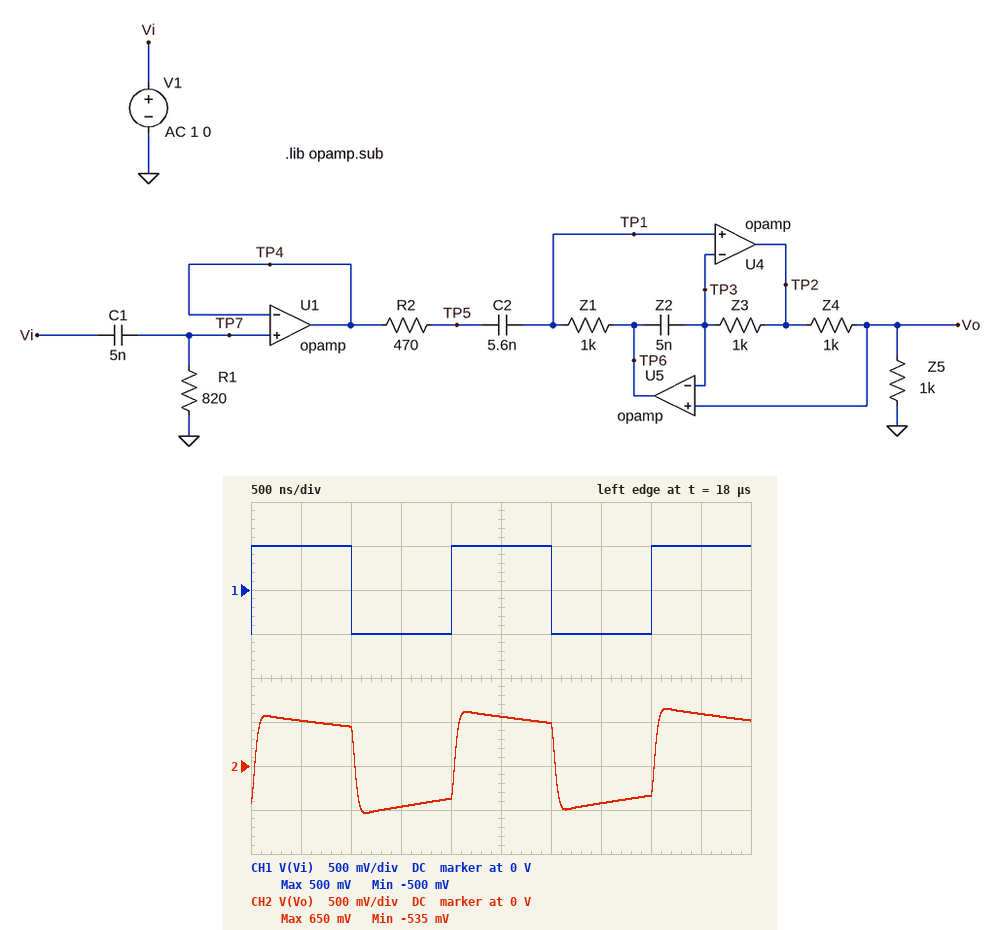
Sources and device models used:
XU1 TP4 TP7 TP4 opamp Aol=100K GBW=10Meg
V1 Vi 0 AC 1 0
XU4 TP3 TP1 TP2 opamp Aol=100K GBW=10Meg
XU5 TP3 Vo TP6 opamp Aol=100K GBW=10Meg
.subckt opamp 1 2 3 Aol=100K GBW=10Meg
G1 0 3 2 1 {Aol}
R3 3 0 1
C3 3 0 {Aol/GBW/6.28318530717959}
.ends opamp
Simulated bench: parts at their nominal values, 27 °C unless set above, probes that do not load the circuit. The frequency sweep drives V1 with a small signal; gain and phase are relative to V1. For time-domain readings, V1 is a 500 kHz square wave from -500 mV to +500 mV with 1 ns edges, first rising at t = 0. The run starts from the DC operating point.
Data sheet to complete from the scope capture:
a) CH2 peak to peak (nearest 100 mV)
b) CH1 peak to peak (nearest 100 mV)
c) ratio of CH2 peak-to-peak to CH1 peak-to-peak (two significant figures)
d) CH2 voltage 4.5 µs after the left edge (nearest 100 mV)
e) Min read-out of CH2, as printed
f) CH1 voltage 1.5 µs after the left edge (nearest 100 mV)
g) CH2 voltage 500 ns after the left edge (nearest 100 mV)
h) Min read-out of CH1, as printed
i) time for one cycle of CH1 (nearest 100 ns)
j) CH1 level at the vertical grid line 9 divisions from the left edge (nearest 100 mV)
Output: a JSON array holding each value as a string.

["1.2 V", "1.0 V", "1.2", "600 mV", "-535 mV", "-500 mV", "500 mV", "-500 mV", "2.0 µs", "500 mV"]
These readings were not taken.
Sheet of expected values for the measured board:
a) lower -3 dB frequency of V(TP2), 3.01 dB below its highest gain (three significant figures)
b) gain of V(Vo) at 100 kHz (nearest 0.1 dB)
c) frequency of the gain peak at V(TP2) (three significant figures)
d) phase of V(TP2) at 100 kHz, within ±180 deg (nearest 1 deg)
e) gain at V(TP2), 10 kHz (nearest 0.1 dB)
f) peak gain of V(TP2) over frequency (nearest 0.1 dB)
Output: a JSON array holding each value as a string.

["26.9 kHz", "0 dB", "33.6 kHz", "29 deg", "-24.3 dB", "8.6 dB"]
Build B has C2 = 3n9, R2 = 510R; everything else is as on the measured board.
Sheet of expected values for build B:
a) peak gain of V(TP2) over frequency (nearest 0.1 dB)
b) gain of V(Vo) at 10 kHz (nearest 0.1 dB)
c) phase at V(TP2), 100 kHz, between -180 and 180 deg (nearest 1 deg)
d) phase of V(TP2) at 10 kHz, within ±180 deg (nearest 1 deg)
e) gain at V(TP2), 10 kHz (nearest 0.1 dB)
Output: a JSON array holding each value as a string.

["10.1 dB", "-33.7 dB", "30 deg", "-112 deg", "-27.7 dB"]
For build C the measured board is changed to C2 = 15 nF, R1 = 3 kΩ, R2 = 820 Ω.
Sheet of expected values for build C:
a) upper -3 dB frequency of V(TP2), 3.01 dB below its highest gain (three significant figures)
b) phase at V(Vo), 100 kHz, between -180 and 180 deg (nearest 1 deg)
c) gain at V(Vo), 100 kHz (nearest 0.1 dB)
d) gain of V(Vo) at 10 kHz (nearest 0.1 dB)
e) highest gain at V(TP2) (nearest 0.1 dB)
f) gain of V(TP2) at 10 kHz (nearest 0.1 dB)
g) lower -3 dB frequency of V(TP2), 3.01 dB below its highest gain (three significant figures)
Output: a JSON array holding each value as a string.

["3.63 MHz", "19 deg", "-0.1 dB", "-14.2 dB", "6.0 dB", "-8.2 dB", "20.9 kHz"]
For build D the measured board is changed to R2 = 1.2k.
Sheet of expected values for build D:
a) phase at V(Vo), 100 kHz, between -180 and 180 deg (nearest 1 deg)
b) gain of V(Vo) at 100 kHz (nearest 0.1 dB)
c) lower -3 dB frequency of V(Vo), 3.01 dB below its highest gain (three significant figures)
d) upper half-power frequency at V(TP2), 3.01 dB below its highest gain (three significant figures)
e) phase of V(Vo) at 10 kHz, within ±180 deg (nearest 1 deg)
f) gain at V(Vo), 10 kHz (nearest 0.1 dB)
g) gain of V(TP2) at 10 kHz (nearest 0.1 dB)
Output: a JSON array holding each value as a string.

["41 deg", "-0.5 dB", "40.8 kHz", "2.93 MHz", "-130 deg", "-31.0 dB", "-25.0 dB"]
